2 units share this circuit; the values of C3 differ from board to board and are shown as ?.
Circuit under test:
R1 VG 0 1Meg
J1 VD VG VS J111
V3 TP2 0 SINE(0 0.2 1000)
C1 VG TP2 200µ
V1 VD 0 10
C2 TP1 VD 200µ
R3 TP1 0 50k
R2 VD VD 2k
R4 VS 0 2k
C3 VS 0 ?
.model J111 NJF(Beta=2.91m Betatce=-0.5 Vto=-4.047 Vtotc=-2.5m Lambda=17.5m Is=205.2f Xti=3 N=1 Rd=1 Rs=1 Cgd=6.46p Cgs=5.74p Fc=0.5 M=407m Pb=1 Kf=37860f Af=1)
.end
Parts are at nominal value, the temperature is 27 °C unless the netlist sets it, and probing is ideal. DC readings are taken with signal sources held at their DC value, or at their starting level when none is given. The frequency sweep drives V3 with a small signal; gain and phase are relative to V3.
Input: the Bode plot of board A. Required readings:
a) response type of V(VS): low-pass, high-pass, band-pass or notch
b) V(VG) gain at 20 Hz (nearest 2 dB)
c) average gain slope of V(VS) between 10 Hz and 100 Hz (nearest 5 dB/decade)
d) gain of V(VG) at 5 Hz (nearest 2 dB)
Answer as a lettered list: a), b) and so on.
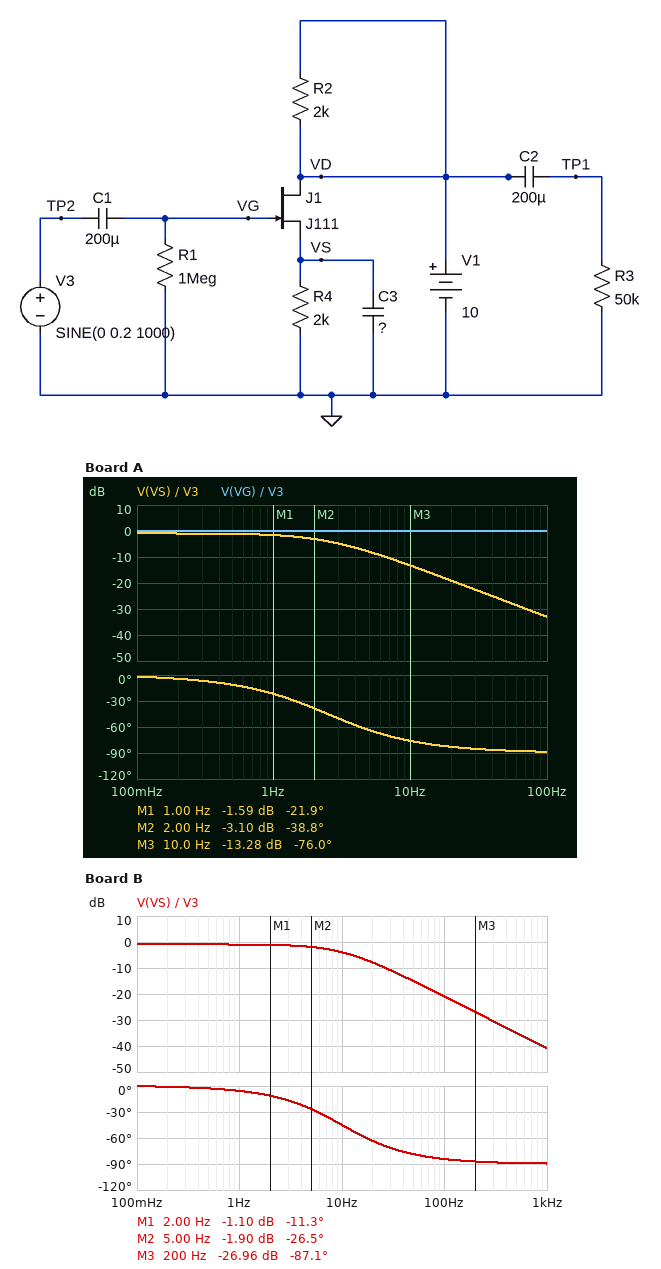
a) low-pass
b) 0 dB
c) -20 dB/decade
d) 0 dB
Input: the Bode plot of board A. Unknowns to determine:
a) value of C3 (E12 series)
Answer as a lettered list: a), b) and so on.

a) 330 µF
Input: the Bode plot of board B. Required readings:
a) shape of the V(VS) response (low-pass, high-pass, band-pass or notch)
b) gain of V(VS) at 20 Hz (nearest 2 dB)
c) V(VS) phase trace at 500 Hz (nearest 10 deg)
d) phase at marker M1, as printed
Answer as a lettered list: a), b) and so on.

a) low-pass
b) -8 dB
c) -90 deg
d) -11.3 deg
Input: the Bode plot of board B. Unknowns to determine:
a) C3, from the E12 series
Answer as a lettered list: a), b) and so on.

a) 82 µF
